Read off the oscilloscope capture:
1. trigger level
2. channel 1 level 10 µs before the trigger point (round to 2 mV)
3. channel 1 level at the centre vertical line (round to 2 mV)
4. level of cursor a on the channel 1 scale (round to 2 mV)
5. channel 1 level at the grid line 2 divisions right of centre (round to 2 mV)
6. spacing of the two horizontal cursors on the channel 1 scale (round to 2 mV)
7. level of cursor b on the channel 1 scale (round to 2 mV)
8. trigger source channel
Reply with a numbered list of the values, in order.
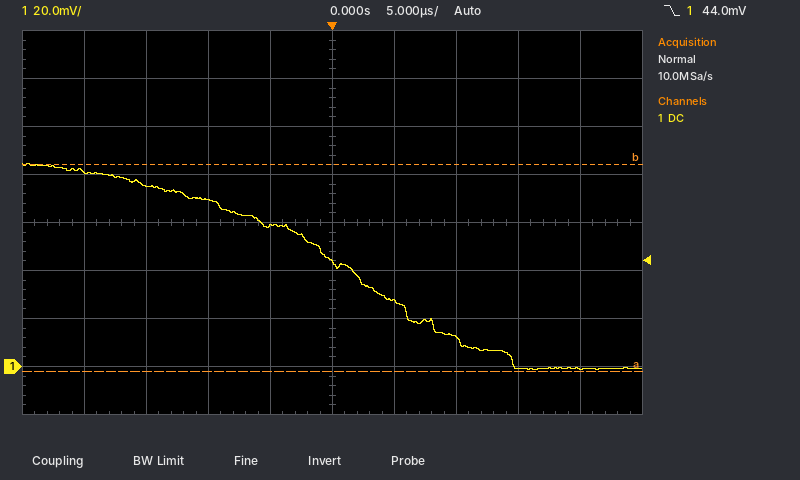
1. 44.0 mV
2. 70 mV
3. 44 mV
4. -2 mV
5. 12 mV
6. 86 mV
7. 84 mV
8. channel 1
